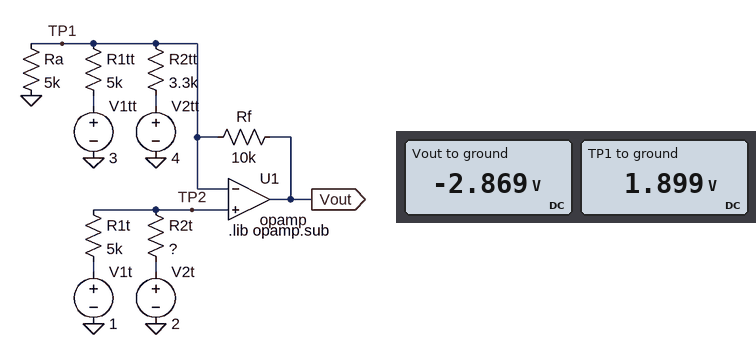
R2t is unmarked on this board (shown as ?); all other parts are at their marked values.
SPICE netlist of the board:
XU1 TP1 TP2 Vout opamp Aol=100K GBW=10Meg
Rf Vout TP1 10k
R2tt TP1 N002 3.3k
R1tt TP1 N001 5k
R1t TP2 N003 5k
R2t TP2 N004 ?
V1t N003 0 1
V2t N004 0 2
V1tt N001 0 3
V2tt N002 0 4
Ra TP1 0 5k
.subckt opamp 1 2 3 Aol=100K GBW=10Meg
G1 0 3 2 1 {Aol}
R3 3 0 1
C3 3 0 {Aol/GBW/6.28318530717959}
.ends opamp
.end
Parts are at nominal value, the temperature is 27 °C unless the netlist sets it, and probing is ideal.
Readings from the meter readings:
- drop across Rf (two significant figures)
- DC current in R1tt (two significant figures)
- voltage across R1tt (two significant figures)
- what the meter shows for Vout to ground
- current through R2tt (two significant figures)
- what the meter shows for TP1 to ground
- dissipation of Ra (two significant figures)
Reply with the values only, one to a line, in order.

4.8 V
220 µA
1.1 V
-2.869 V
640 µA
1.899 V
720 µW
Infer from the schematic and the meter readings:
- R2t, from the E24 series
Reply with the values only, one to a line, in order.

560 Ω
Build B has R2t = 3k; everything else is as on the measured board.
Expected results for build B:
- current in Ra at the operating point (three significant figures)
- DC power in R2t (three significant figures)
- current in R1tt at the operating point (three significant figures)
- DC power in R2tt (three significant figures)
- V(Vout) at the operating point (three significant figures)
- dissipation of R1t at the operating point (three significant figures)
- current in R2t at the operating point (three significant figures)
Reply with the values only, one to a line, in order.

325 µA
46.9 µW
275 µA
1.71 mW
-5.07 V
78.1 µW
125 µA
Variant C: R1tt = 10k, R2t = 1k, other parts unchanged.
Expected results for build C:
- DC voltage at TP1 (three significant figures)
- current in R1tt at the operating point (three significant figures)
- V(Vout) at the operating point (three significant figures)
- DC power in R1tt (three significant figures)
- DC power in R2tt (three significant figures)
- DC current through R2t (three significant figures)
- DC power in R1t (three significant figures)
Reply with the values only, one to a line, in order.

1.83 V
117 µA
-2.23 V
136 µW
1.42 mW
167 µA
139 µW
